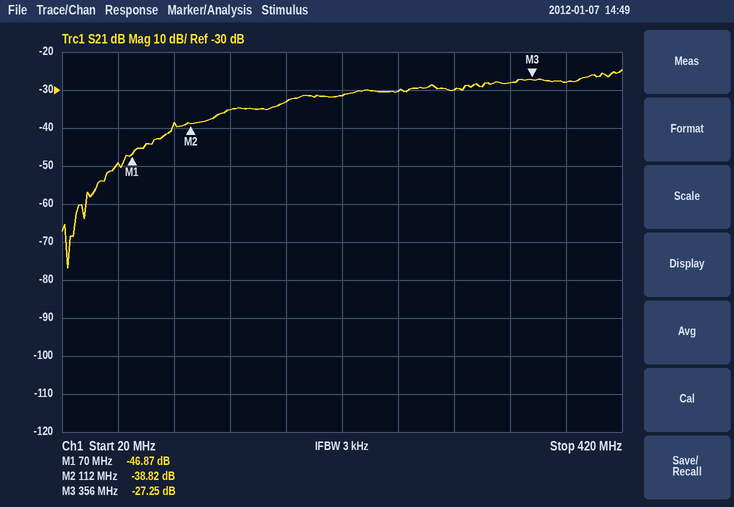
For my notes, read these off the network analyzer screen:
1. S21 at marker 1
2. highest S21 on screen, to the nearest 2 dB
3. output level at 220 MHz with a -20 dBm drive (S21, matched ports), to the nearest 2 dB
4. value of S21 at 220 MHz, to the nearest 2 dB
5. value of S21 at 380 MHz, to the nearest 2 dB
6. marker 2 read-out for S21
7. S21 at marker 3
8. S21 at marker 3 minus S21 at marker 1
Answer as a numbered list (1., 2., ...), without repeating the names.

1. -46.87 dB
2. -24 dB
3. -52 dBm
4. -32 dB
5. -28 dB
6. -38.82 dB
7. -27.25 dB
8. 19.62 dB
